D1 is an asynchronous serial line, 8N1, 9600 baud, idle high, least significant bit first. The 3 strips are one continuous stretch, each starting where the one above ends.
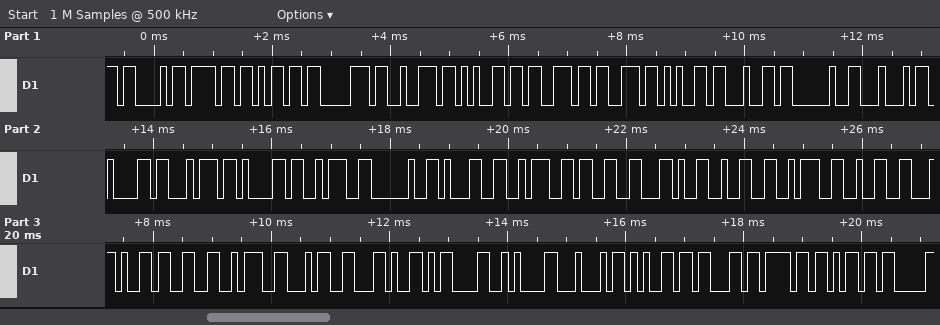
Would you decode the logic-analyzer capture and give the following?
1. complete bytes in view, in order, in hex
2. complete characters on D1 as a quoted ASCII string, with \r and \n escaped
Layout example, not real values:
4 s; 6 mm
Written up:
43 6F 6D 70 72 65 73 73 65 64 20 44 61 74 61 3A 20 31 3A 33 2C 32 3A 32 2C 33 3A 34 2C 0D 0A 44 65 63 6F 6D; "Compressed Data: 1:3,2:2,3:4,\r\nDecom"
